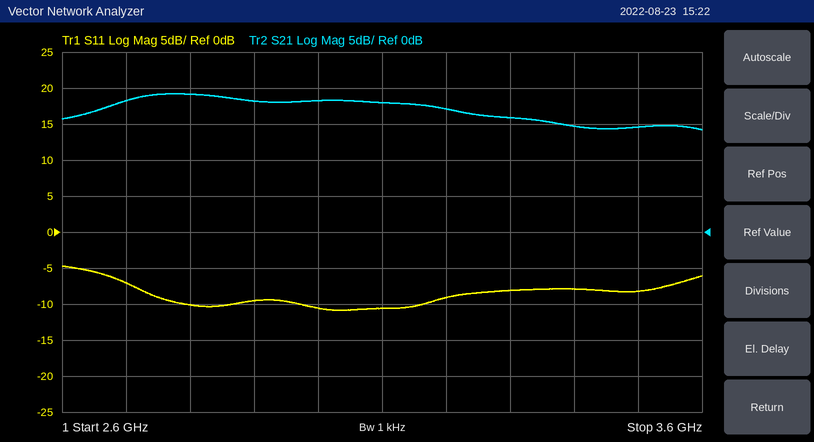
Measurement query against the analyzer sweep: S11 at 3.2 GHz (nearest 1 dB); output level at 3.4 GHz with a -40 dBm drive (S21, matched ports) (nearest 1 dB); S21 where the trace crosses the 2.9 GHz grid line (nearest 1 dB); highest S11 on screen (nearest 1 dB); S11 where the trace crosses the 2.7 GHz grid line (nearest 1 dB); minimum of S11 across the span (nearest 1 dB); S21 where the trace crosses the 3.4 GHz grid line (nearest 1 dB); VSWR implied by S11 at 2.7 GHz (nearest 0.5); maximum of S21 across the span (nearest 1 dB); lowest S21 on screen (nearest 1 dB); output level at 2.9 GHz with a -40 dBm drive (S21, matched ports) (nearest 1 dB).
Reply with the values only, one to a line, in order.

-9 dB
-25 dBm
18 dB
-5 dB
-7 dB
-11 dB
15 dB
2.5
19 dB
14 dB
-22 dBm
